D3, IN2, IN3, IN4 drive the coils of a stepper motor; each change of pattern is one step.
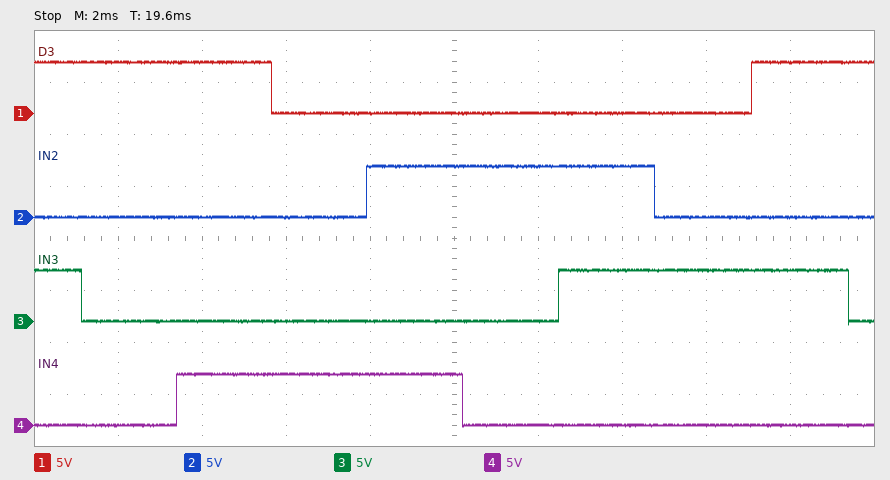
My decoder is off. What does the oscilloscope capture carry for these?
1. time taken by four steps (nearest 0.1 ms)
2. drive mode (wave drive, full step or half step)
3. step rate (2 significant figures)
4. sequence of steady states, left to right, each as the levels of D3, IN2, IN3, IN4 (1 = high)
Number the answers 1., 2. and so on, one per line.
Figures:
1. 9.1 ms
2. half step
3. 440 steps/s
4. 1010 1000 1001 0001 0101 0100 0110 0010 1010 1000
